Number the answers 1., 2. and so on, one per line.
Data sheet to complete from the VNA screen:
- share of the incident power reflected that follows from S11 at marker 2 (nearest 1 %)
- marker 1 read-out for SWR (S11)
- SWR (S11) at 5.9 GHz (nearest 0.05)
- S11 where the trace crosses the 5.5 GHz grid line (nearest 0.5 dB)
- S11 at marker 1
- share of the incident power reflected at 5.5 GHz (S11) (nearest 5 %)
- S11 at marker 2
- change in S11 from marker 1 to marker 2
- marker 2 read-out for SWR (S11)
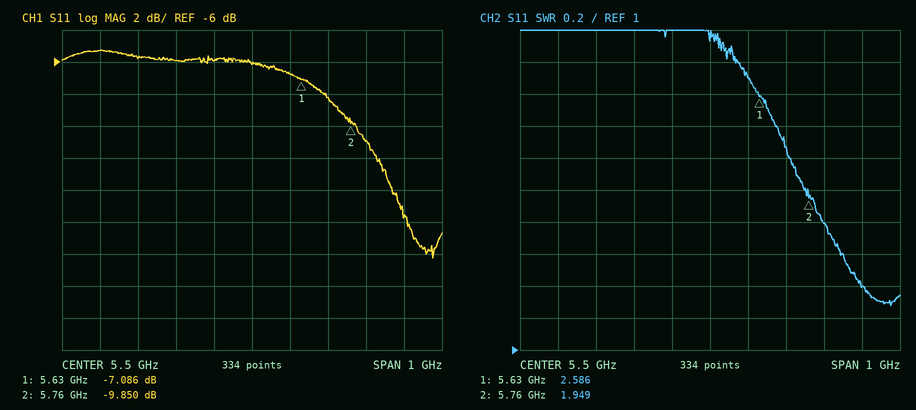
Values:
1. 10 %
2. 2.586
3. 1.40
4. -6.0 dB
5. -7.086 dB
6. 25 %
7. -9.850 dB
8. -2.764 dB
9. 1.949
